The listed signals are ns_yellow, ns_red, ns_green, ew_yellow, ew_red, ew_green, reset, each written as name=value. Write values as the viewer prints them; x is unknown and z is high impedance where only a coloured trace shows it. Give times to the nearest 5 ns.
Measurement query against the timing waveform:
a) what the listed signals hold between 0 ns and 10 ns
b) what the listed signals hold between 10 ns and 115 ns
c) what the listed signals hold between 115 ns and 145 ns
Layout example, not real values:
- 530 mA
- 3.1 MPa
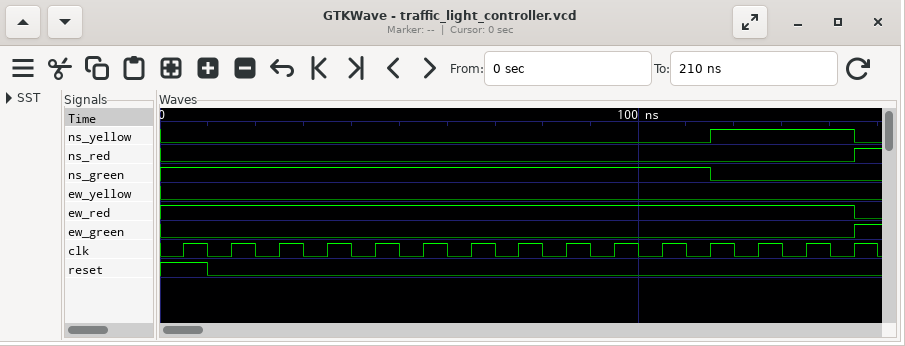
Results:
- ns_yellow=0, ns_red=0, ns_green=1, ew_yellow=0, ew_red=1, ew_green=0, reset=1
- ns_yellow=0, ns_red=0, ns_green=1, ew_yellow=0, ew_red=1, ew_green=0, reset=0
- ns_yellow=1, ns_red=0, ns_green=0, ew_yellow=0, ew_red=1, ew_green=0, reset=0
